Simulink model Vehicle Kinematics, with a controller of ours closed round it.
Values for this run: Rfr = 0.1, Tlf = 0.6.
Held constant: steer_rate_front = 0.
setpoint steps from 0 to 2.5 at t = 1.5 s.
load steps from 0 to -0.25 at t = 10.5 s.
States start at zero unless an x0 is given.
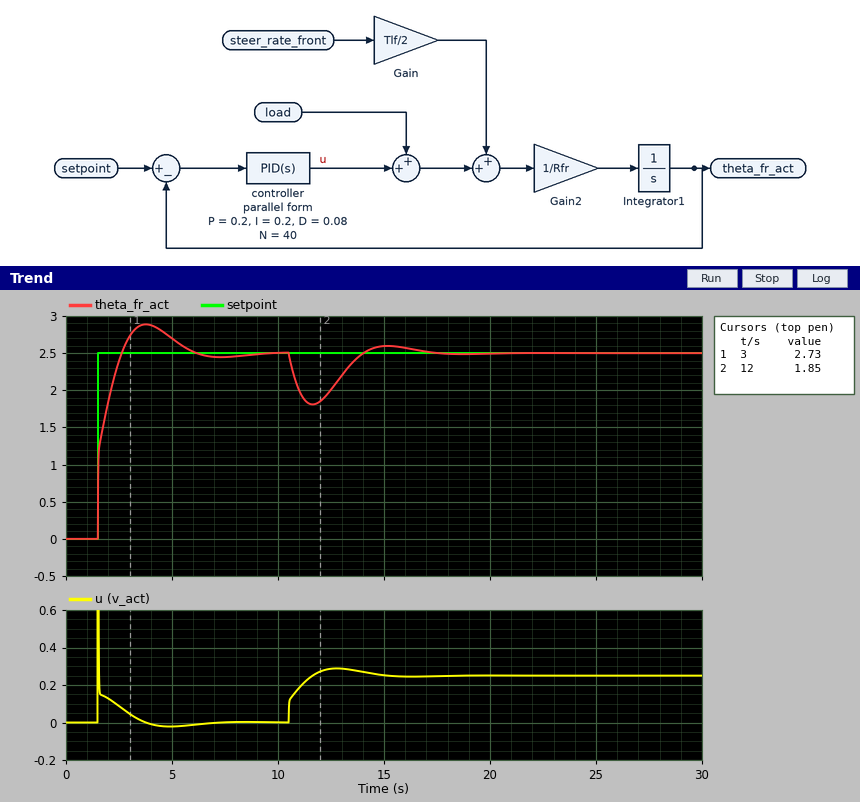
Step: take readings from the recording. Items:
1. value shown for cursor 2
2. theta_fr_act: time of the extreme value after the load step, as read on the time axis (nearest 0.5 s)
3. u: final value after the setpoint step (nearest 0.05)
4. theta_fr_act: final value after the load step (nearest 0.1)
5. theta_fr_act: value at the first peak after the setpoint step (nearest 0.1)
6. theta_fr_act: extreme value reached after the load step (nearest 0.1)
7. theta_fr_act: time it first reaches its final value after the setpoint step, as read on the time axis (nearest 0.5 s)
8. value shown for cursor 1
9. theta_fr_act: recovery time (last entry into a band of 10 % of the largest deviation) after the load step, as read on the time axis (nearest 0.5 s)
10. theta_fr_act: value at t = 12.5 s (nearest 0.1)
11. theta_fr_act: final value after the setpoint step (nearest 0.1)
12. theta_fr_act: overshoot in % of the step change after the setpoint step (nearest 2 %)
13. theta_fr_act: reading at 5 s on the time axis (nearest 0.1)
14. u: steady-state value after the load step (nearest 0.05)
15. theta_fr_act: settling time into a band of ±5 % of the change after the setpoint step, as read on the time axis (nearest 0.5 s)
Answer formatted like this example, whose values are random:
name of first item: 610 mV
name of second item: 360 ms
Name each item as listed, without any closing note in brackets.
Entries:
value shown for cursor 2: 1.85
theta_fr_act: time of the extreme value after the load step, as read on the time axis: 11.5 s
u: final value after the setpoint step: 0.00
theta_fr_act: final value after the load step: 2.5
theta_fr_act: value at the first peak after the setpoint step: 2.9
theta_fr_act: extreme value reached after the load step: 1.8
theta_fr_act: time it first reaches its final value after the setpoint step, as read on the time axis: 2.5 s
value shown for cursor 1: 2.73
theta_fr_act: recovery time (last entry into a band of 10 % of the largest deviation) after the load step, as read on the time axis: 16.0 s
theta_fr_act: value at t = 12.5 s: 2.0
theta_fr_act: final value after the setpoint step: 2.5
theta_fr_act: overshoot in % of the step change after the setpoint step: 16 %
theta_fr_act: reading at 5 s on the time axis: 2.7
u: steady-state value after the load step: 0.25
theta_fr_act: settling time into a band of ±5 % of the change after the setpoint step, as read on the time axis: 5.5 s
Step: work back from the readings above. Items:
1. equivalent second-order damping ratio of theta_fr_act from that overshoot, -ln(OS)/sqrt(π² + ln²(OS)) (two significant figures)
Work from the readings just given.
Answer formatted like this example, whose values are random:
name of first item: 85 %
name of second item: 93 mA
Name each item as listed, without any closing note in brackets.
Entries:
equivalent second-order damping ratio of theta_fr_act from that overshoot, -ln(OS)/sqrt(π² + ln²(OS)): 0.50
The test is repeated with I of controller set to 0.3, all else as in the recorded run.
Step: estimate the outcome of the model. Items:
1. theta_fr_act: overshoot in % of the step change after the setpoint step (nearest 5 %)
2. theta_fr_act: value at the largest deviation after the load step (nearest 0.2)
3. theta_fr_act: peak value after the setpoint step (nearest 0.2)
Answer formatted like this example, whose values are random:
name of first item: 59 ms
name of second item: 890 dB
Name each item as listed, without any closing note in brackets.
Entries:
theta_fr_act: overshoot in % of the step change after the setpoint step: 20 %
theta_fr_act: value at the largest deviation after the load step: 1.8
theta_fr_act: peak value after the setpoint step: 3.0
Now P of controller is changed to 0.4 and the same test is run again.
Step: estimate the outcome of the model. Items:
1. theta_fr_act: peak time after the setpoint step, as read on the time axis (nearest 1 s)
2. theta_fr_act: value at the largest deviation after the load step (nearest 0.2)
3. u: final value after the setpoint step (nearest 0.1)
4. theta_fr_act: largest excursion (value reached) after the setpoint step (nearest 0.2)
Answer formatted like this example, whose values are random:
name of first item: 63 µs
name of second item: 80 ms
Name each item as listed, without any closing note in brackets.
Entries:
theta_fr_act: peak time after the setpoint step, as read on the time axis: 3 s
theta_fr_act: value at the largest deviation after the load step: 2.0
u: final value after the setpoint step: 0.0
theta_fr_act: largest excursion (value reached) after the setpoint step: 2.6
